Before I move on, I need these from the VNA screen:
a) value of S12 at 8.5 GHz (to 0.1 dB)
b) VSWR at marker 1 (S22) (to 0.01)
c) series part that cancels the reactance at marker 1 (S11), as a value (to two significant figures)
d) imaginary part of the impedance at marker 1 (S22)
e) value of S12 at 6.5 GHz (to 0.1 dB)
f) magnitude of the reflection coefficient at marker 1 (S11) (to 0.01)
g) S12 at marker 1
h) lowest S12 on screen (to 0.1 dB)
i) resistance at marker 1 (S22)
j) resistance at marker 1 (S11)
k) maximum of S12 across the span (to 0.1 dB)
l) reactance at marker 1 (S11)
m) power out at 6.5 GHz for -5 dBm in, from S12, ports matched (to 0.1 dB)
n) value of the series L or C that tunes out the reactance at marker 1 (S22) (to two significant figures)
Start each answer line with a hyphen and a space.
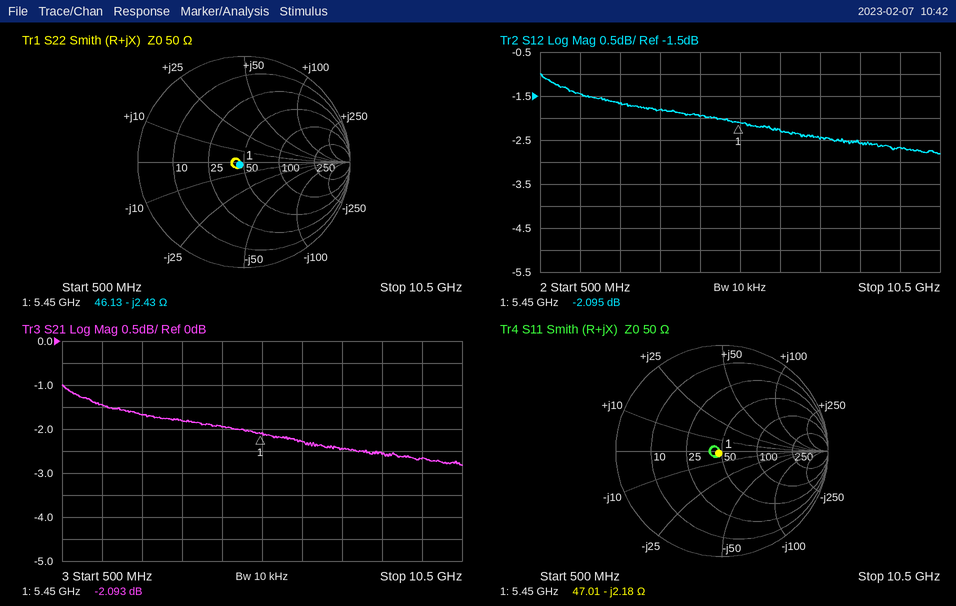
- -2.6 dB
- 1.10
- 64 pH
- -2.43 Ω
- -2.3 dB
- 0.04
- -2.095 dB
- -2.8 dB
- 46.13 Ω
- 47.01 Ω
- -1.0 dB
- -2.18 Ω
- -7.3 dBm
- 71 pH
